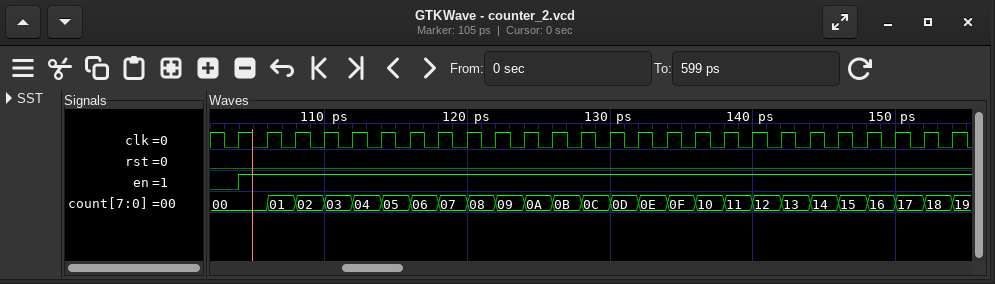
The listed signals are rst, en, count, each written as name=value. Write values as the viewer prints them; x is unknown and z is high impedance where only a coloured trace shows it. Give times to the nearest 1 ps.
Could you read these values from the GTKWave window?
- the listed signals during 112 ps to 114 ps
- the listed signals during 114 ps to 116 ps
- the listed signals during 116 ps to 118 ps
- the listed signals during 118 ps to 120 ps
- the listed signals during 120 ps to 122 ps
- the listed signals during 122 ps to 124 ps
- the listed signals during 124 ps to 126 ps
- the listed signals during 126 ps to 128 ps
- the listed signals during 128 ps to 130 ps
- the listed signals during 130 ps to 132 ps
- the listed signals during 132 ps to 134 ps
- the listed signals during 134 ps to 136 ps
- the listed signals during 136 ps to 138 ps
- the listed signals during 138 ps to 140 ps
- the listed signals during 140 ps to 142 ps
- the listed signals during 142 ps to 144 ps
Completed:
rst=0, en=1, count=04
rst=0, en=1, count=05
rst=0, en=1, count=06
rst=0, en=1, count=07
rst=0, en=1, count=08
rst=0, en=1, count=09
rst=0, en=1, count=0A
rst=0, en=1, count=0B
rst=0, en=1, count=0C
rst=0, en=1, count=0D
rst=0, en=1, count=0E
rst=0, en=1, count=0F
rst=0, en=1, count=10
rst=0, en=1, count=11
rst=0, en=1, count=12
rst=0, en=1, count=13
